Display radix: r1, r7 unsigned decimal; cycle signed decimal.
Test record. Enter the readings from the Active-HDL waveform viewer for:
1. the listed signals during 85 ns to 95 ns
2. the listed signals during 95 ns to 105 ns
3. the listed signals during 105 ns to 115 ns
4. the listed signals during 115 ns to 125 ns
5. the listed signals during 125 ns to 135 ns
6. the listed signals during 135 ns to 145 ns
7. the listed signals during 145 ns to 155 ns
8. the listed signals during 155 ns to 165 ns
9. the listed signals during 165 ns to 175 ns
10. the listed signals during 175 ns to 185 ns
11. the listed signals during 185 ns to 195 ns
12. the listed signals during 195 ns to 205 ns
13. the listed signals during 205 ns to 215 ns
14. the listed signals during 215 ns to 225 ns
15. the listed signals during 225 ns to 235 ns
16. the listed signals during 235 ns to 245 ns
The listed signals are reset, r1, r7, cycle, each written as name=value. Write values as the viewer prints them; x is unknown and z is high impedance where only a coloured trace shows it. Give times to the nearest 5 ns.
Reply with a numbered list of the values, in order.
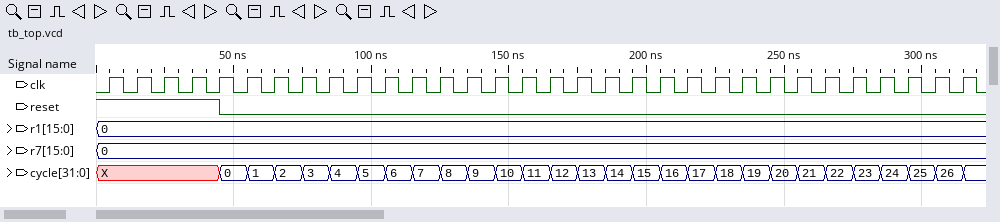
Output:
1. reset=0, r1=0, r7=0, cycle=4
2. reset=0, r1=0, r7=0, cycle=5
3. reset=0, r1=0, r7=0, cycle=6
4. reset=0, r1=0, r7=0, cycle=7
5. reset=0, r1=0, r7=0, cycle=8
6. reset=0, r1=0, r7=0, cycle=9
7. reset=0, r1=0, r7=0, cycle=10
8. reset=0, r1=0, r7=0, cycle=11
9. reset=0, r1=0, r7=0, cycle=12
10. reset=0, r1=0, r7=0, cycle=13
11. reset=0, r1=0, r7=0, cycle=14
12. reset=0, r1=0, r7=0, cycle=15
13. reset=0, r1=0, r7=0, cycle=16
14. reset=0, r1=0, r7=0, cycle=17
15. reset=0, r1=0, r7=0, cycle=18
16. reset=0, r1=0, r7=0, cycle=19
